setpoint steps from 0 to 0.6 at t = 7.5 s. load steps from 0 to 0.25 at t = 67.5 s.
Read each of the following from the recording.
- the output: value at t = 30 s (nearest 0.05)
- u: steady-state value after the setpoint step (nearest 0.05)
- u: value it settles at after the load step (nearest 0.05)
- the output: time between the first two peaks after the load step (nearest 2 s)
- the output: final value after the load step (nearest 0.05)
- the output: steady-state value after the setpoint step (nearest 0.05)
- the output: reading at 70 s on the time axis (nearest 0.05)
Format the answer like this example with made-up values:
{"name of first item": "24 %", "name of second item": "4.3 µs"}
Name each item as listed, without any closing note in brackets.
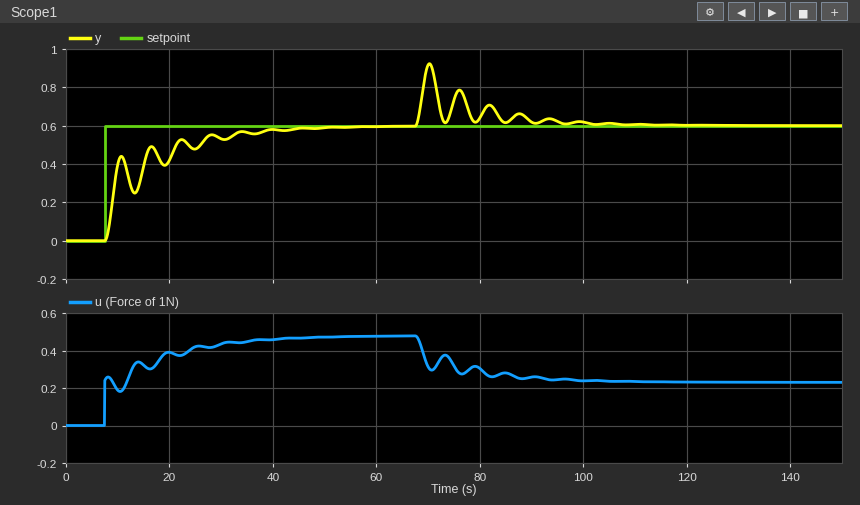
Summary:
{"the output: value at t = 30 s": "0.55", "u: steady-state value after the setpoint step": "0.50", "u: value it settles at after the load step": "0.25", "the output: time between the first two peaks after the load step": "6 s", "the output: final value after the load step": "0.60", "the output: steady-state value after the setpoint step": "0.60", "the output: reading at 70 s on the time axis": "0.90"}
